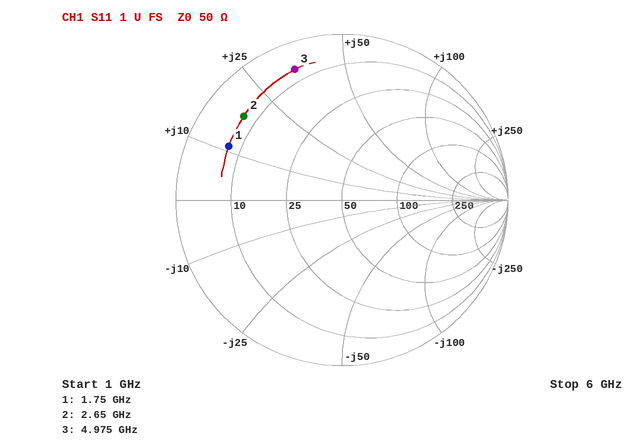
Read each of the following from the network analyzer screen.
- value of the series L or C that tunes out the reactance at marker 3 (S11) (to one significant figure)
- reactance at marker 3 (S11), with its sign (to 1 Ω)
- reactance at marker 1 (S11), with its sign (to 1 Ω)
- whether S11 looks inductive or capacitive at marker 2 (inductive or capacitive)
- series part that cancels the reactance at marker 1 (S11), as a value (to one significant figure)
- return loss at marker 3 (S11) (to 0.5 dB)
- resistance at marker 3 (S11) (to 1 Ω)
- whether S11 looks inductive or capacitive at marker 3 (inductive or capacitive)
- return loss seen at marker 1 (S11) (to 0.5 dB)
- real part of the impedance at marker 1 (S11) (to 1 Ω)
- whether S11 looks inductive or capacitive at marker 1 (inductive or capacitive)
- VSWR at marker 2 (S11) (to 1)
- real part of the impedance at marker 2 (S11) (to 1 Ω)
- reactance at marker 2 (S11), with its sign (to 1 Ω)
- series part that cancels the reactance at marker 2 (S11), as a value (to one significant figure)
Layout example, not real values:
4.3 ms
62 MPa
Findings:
900 fF
+35 Ω
+11 Ω
inductive
8 pF
1.5 dB
7 Ω
inductive
2.5 dB
7 Ω
inductive
8
7 Ω
+18 Ω
3 pF
